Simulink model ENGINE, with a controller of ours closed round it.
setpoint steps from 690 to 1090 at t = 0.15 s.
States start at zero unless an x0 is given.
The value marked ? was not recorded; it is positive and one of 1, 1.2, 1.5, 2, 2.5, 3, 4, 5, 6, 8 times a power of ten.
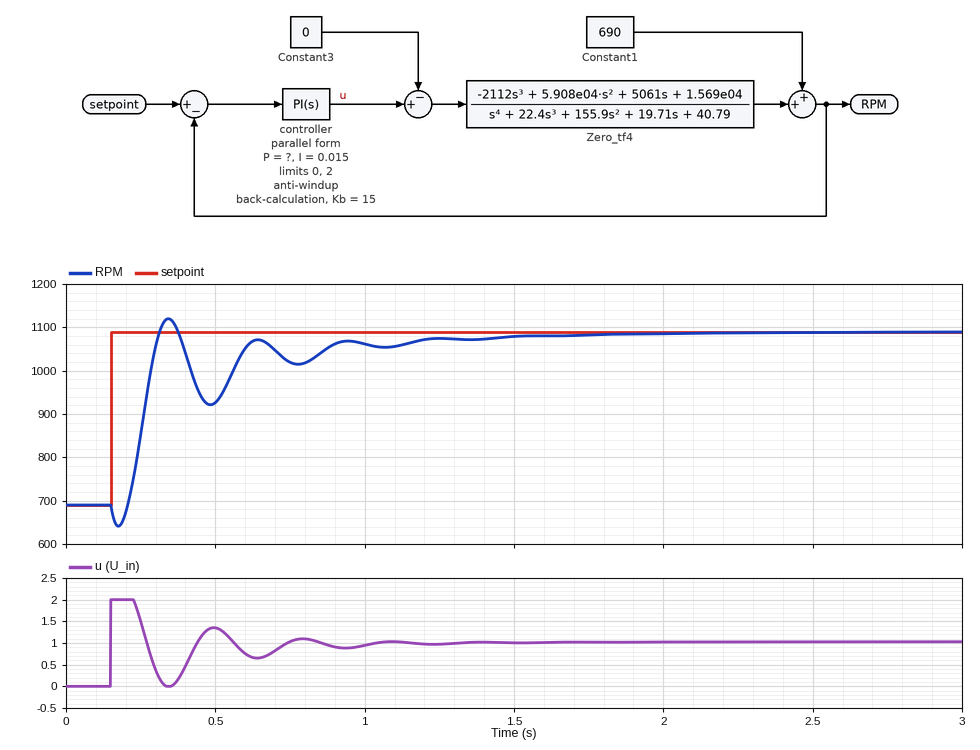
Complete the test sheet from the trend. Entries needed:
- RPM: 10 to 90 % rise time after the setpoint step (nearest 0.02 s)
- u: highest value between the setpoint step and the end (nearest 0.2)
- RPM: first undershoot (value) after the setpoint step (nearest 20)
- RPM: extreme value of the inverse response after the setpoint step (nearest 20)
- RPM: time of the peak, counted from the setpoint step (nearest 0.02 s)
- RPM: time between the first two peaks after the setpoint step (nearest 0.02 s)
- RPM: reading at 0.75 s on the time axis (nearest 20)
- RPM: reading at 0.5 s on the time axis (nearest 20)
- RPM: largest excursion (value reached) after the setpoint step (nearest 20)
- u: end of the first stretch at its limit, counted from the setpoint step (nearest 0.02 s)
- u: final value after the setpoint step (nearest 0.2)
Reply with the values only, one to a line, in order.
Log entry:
0.08 s
2.0
920
640
0.20 s
0.30 s
1020
920
1120
0.08 s
1.0
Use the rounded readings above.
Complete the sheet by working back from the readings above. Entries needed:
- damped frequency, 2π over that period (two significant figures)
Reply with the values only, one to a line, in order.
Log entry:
21 rad/s
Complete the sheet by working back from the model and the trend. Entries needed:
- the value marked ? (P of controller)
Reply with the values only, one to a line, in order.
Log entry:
0.006
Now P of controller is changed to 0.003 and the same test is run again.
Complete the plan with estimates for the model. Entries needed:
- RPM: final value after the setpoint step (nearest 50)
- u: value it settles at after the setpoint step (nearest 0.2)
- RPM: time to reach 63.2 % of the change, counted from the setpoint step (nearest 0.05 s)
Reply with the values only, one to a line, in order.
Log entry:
1100
1.0
0.15 s
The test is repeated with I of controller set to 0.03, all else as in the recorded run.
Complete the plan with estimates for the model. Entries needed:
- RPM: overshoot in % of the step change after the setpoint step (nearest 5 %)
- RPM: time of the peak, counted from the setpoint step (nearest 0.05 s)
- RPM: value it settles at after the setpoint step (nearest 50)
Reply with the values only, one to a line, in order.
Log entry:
20 %
0.20 s
1100
